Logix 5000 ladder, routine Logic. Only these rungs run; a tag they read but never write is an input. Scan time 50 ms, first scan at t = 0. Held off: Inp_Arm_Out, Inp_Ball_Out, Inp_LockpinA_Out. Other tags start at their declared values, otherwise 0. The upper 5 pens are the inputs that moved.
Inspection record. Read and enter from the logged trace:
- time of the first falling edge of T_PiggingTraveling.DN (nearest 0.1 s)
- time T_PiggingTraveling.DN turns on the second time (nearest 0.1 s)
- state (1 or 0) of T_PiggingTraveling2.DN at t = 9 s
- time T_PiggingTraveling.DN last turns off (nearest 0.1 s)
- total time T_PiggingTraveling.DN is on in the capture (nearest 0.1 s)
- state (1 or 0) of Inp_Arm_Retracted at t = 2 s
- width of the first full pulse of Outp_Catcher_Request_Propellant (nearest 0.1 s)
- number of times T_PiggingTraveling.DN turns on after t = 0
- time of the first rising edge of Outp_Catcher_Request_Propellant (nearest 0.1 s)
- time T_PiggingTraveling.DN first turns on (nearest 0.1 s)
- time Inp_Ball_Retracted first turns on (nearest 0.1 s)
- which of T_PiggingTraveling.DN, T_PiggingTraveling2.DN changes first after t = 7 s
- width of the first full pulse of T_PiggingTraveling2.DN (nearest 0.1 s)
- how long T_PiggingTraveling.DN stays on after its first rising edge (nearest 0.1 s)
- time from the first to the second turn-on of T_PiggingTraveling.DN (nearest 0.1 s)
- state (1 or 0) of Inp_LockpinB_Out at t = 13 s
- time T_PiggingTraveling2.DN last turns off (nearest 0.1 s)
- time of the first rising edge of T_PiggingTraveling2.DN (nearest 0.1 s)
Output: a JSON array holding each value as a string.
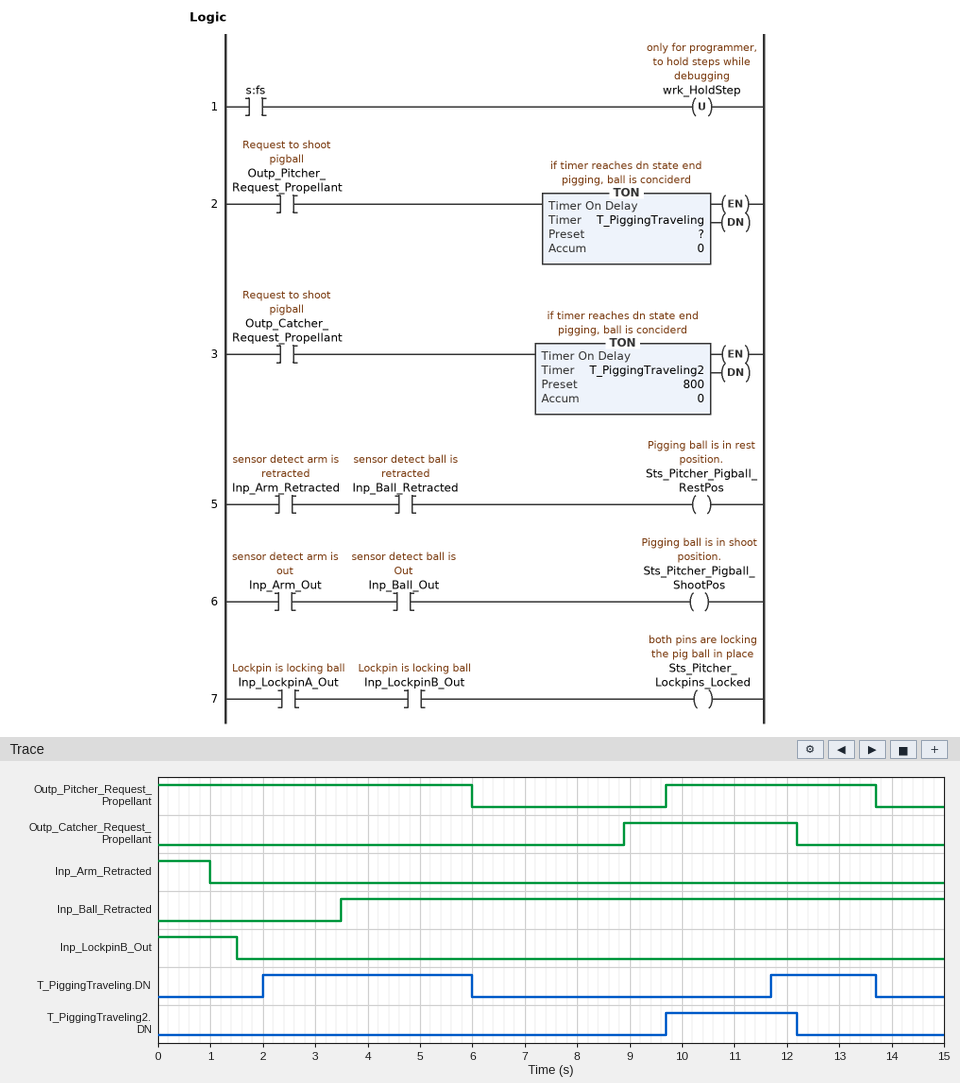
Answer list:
["6.0 s", "11.7 s", "0", "13.7 s", "6.0 s", "0", "3.3 s", "2", "8.9 s", "2.0 s", "3.5 s", "T_PiggingTraveling2.DN", "2.5 s", "4.0 s", "9.7 s", "0", "12.2 s", "9.7 s"]
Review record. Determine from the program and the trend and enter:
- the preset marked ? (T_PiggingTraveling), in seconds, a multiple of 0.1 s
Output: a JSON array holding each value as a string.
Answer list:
["2.0 s"]
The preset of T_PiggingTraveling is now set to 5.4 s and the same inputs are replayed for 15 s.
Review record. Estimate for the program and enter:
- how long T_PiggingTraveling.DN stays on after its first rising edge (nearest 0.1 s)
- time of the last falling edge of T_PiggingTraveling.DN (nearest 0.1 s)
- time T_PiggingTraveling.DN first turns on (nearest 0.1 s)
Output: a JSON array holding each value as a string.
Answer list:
["0.6 s", "6.0 s", "5.4 s"]
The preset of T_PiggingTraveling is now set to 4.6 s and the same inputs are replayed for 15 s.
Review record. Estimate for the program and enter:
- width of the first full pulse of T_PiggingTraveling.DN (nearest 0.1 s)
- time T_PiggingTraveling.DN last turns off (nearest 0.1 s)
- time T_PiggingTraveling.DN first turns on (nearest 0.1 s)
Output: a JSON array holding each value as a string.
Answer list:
["1.4 s", "6.0 s", "4.6 s"]
